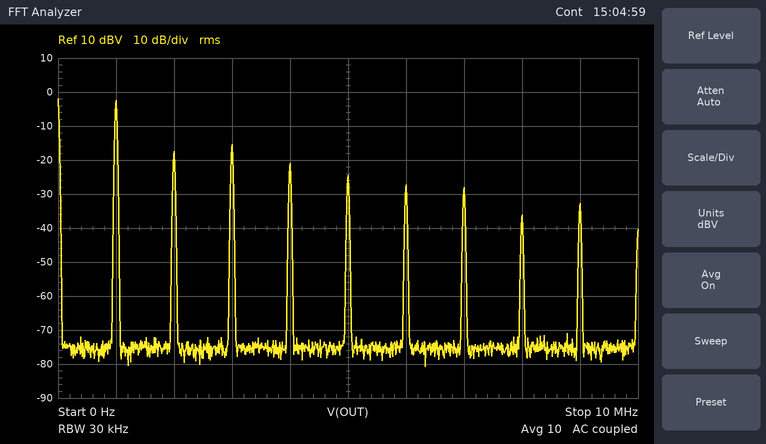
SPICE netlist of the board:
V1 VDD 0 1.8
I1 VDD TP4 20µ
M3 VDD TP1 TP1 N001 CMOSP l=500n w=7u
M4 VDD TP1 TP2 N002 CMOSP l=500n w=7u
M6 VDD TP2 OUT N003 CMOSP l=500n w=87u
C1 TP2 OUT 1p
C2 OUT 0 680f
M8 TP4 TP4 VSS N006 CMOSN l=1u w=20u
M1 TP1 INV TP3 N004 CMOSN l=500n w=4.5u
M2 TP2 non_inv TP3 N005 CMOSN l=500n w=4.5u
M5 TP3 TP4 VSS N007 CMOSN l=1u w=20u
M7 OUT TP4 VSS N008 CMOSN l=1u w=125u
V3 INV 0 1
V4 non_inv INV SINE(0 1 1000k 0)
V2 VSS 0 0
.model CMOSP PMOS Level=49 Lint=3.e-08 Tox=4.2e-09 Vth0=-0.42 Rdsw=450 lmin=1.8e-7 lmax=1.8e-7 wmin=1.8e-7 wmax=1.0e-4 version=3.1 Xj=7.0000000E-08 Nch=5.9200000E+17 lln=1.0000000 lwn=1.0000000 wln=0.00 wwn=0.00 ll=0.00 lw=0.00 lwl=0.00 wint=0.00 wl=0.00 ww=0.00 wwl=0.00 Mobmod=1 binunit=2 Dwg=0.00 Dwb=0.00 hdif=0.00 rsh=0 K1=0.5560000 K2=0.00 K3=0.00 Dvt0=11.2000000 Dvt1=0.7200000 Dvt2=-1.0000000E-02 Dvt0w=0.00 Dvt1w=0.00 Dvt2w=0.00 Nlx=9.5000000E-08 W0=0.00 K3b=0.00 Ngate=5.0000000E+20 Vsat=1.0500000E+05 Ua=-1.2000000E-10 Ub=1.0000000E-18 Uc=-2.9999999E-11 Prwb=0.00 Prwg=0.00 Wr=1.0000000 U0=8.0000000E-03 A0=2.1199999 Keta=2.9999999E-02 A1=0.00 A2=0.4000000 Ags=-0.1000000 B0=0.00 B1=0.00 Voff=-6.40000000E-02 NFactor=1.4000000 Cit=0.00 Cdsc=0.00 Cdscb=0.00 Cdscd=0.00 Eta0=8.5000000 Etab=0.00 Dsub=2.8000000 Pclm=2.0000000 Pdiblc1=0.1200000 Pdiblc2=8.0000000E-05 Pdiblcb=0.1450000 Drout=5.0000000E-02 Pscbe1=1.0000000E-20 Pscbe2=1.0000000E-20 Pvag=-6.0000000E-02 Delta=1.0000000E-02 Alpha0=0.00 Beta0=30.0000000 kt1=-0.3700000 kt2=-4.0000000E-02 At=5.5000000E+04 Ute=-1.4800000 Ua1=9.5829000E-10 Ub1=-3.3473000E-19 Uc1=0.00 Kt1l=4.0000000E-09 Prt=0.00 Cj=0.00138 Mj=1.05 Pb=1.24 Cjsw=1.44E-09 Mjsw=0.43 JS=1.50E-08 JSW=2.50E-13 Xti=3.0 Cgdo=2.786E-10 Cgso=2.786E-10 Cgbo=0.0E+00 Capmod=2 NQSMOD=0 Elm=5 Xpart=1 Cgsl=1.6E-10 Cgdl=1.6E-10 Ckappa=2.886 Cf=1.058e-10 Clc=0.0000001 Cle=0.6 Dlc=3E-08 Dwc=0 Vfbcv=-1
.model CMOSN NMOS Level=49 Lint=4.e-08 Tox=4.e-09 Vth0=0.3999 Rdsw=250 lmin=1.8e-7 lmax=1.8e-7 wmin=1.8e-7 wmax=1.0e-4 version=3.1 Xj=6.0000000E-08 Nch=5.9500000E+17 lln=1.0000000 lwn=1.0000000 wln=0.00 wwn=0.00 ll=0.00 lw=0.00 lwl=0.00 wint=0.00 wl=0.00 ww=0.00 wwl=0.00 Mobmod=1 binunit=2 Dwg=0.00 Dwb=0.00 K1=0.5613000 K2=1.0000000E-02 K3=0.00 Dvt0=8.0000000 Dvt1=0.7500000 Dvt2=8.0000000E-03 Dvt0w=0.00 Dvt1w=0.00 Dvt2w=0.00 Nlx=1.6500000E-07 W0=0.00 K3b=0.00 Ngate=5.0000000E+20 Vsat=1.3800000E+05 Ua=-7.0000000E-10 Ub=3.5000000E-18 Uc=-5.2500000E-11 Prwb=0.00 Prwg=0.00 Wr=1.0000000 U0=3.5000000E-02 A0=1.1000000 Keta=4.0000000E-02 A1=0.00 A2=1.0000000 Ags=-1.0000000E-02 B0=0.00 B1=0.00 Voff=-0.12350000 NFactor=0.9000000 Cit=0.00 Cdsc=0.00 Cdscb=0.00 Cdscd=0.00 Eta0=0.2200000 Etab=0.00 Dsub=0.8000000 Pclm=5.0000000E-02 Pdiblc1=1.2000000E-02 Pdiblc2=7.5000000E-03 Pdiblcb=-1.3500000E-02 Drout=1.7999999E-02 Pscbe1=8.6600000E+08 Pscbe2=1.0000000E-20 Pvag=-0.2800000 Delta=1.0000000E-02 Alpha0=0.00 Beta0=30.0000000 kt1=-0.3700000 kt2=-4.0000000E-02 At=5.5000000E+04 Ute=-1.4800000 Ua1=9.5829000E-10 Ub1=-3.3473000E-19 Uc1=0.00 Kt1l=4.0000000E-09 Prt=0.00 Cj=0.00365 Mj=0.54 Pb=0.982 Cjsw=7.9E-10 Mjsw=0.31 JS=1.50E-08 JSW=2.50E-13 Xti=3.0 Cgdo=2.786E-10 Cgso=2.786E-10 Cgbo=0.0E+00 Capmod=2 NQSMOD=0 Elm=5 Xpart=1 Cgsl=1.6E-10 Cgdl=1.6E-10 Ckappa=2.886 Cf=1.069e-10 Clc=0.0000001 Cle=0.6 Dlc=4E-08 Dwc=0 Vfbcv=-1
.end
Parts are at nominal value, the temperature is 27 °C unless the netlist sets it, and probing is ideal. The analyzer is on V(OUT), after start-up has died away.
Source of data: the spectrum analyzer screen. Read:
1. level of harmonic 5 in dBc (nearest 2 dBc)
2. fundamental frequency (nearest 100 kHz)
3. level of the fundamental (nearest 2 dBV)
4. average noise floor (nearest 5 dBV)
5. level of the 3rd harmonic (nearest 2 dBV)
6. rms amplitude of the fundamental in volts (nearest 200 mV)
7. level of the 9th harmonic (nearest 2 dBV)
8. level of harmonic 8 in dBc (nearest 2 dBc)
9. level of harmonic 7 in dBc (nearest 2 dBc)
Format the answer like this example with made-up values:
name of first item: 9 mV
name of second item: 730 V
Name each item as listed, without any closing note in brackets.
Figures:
level of harmonic 5 in dBc: -22 dBc
fundamental frequency: 1.0 MHz
level of the fundamental: -2 dBV
average noise floor: -75 dBV
level of the 3rd harmonic: -16 dBV
rms amplitude of the fundamental in volts: 800 mV
level of the 9th harmonic: -32 dBV
level of harmonic 8 in dBc: -34 dBc
level of harmonic 7 in dBc: -26 dBc
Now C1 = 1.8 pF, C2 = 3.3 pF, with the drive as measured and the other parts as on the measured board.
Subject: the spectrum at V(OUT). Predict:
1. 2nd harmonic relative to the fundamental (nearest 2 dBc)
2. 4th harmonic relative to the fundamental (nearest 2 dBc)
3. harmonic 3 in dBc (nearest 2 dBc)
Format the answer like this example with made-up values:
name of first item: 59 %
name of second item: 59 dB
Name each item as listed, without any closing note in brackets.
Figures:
2nd harmonic relative to the fundamental: -12 dBc
4th harmonic relative to the fundamental: -22 dBc
harmonic 3 in dBc: -16 dBc
